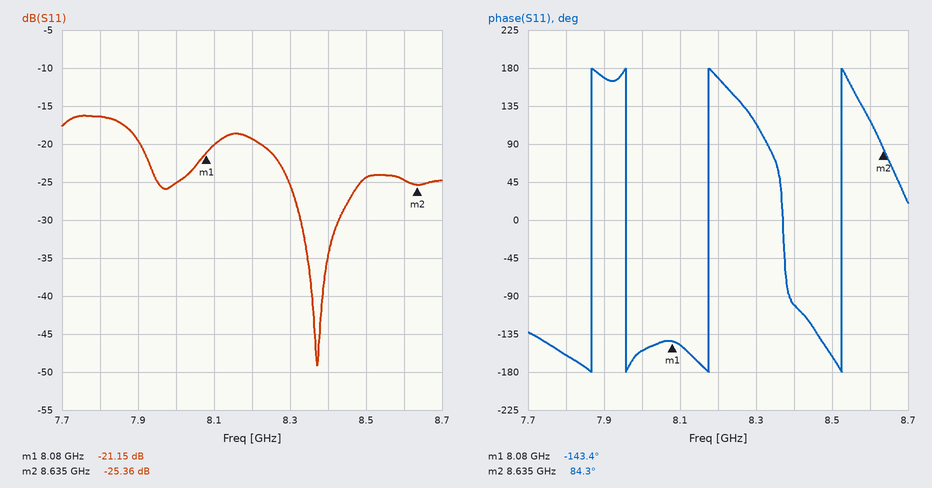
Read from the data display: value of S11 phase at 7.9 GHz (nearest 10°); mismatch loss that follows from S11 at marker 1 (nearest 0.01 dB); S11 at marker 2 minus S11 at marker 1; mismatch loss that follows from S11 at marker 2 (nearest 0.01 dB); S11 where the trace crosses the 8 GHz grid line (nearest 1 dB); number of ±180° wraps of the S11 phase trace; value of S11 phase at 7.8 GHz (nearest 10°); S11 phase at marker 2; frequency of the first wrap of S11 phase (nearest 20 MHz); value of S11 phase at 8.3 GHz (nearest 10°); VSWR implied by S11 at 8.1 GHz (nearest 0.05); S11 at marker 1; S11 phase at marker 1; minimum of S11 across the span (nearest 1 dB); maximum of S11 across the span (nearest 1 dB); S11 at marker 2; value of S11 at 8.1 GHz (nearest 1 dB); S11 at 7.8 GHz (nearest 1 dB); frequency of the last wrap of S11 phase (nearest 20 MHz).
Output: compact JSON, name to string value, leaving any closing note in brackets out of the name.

{"value of S11 phase at 7.9 GHz": "170°", "mismatch loss that follows from S11 at marker 1": "0.03 dB", "S11 at marker 2 minus S11 at marker 1": "-4.21 dB", "mismatch loss that follows from S11 at marker 2": "0.01 dB", "S11 where the trace crosses the 8 GHz grid line": "-25 dB", "number of ±180° wraps of the S11 phase trace": "4", "value of S11 phase at 7.8 GHz": "-160°", "S11 phase at marker 2": "84.3°", "frequency of the first wrap of S11 phase": "7.86 GHz", "value of S11 phase at 8.3 GHz": "110°", "VSWR implied by S11 at 8.1 GHz": "1.20", "S11 at marker 1": "-21.15 dB", "S11 phase at marker 1": "-143.4°", "minimum of S11 across the span": "-49 dB", "maximum of S11 across the span": "-16 dB", "S11 at marker 2": "-25.36 dB", "value of S11 at 8.1 GHz": "-20 dB", "S11 at 7.8 GHz": "-16 dB", "frequency of the last wrap of S11 phase": "8.52 GHz"}
